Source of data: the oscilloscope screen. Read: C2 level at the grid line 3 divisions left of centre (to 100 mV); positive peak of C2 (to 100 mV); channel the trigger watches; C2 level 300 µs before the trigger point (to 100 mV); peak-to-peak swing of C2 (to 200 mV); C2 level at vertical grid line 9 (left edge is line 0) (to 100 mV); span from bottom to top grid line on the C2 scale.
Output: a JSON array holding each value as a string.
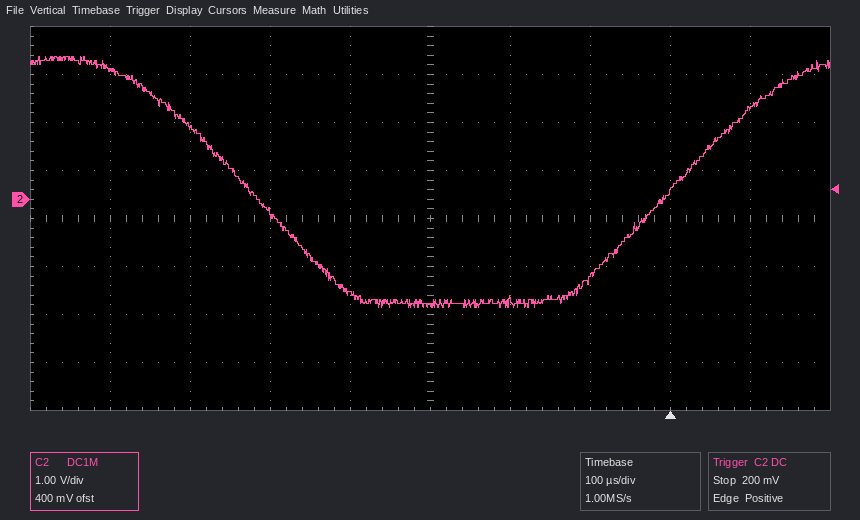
["1.5 V", "3.0 V", "C2", "-2.2 V", "5.2 V", "1.9 V", "8 V"]
